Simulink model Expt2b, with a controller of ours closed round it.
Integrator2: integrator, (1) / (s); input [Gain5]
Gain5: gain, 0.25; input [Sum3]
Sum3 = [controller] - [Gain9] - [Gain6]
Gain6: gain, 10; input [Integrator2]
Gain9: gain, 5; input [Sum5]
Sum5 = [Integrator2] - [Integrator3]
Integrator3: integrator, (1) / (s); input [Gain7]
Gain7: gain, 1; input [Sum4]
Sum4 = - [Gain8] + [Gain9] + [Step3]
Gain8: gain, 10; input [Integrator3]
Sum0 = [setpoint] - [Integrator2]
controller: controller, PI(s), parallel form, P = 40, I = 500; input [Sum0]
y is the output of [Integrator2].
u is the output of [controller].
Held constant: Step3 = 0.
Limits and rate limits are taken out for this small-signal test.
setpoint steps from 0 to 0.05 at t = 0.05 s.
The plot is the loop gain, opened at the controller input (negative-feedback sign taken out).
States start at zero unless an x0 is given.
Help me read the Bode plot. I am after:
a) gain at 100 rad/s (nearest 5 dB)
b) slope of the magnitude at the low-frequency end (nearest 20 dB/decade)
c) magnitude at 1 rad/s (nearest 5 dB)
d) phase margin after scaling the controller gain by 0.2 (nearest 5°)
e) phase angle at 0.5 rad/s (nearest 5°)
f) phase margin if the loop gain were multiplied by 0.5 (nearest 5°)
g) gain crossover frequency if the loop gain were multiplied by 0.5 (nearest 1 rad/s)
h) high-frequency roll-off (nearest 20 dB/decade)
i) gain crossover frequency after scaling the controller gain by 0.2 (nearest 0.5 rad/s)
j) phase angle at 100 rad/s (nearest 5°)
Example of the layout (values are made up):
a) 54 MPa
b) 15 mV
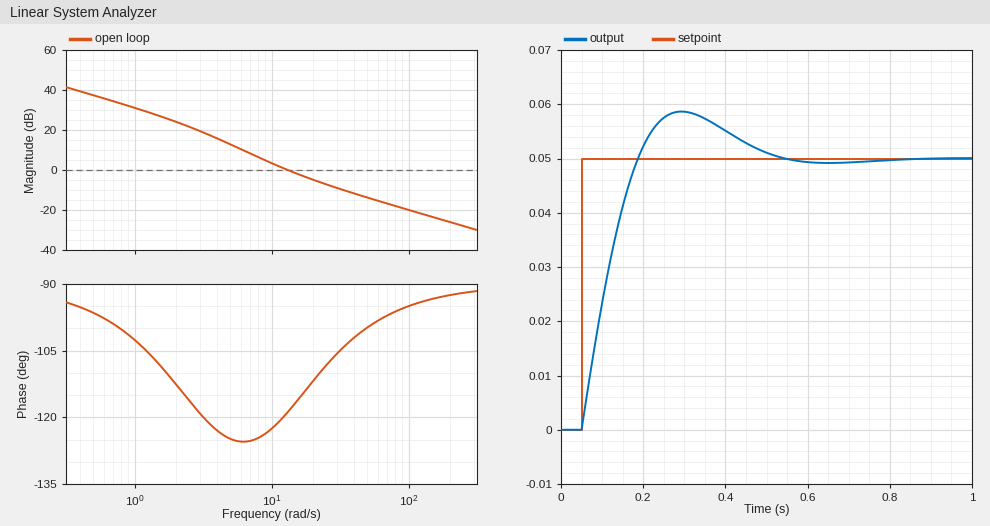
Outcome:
a) -20 dB
b) -20 dB/decade
c) 30 dB
d) 55°
e) -95°
f) 55°
g) 8 rad/s
h) -20 dB/decade
i) 4.5 rad/s
j) -95°
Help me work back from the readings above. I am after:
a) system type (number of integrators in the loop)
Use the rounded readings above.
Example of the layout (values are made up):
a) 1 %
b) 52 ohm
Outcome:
a) 1
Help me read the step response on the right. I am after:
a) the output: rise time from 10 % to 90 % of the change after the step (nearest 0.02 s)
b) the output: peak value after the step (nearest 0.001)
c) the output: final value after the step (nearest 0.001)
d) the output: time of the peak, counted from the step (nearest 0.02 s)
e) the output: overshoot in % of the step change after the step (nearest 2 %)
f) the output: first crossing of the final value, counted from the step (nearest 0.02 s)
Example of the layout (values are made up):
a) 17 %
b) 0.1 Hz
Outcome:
a) 0.10 s
b) 0.059
c) 0.050
d) 0.24 s
e) 18 %
f) 0.14 s
